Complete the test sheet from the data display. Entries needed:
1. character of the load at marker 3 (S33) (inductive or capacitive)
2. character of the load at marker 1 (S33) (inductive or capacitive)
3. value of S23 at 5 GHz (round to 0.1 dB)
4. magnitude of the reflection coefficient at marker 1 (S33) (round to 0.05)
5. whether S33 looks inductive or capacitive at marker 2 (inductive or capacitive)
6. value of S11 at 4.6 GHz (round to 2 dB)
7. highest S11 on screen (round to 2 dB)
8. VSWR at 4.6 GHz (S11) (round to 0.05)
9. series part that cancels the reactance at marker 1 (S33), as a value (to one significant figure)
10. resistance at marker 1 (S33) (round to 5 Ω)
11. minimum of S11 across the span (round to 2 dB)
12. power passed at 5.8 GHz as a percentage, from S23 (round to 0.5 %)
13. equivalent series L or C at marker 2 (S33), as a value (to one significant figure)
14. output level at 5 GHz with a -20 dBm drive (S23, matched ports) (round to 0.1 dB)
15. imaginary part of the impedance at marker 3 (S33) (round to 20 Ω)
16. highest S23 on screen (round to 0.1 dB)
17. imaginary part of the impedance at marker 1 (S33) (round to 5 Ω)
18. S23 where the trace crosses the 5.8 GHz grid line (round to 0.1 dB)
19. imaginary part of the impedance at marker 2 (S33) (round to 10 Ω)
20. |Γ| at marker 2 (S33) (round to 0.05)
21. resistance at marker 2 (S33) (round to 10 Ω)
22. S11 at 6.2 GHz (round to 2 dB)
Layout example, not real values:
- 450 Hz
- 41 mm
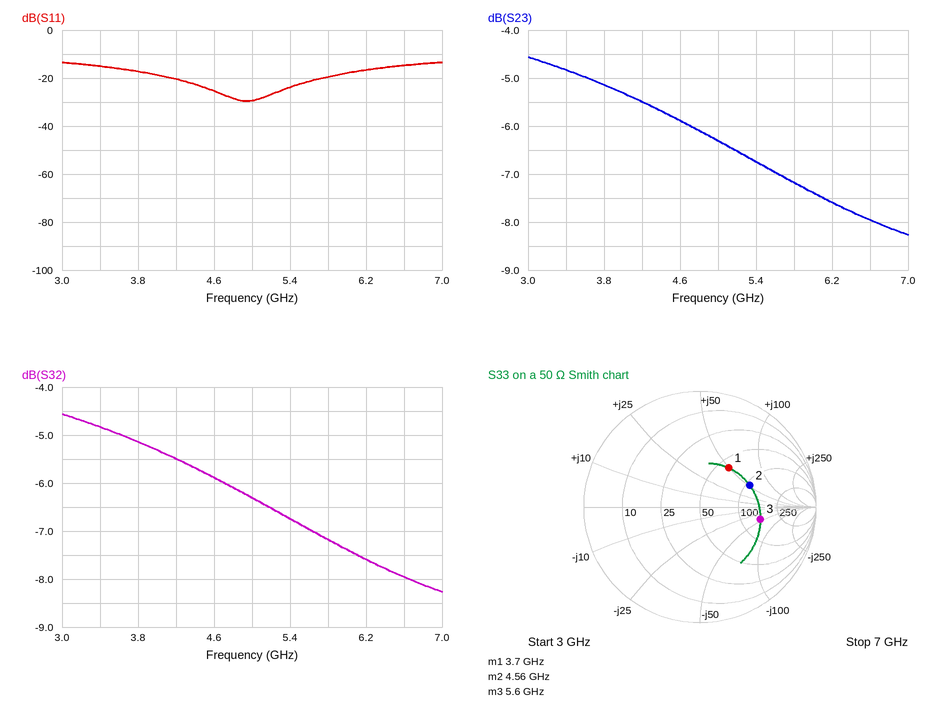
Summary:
- capacitive
- inductive
- -6.3 dB
- 0.40
- inductive
- -26 dB
- -14 dB
- 1.10
- 900 fF
- 60 Ω
- -30 dB
- 19.0 %
- 2 nH
- -26.3 dBm
- -40 Ω
- -4.6 dB
- +50 Ω
- -7.2 dB
- +50 Ω
- 0.45
- 110 Ω
- -16 dB
